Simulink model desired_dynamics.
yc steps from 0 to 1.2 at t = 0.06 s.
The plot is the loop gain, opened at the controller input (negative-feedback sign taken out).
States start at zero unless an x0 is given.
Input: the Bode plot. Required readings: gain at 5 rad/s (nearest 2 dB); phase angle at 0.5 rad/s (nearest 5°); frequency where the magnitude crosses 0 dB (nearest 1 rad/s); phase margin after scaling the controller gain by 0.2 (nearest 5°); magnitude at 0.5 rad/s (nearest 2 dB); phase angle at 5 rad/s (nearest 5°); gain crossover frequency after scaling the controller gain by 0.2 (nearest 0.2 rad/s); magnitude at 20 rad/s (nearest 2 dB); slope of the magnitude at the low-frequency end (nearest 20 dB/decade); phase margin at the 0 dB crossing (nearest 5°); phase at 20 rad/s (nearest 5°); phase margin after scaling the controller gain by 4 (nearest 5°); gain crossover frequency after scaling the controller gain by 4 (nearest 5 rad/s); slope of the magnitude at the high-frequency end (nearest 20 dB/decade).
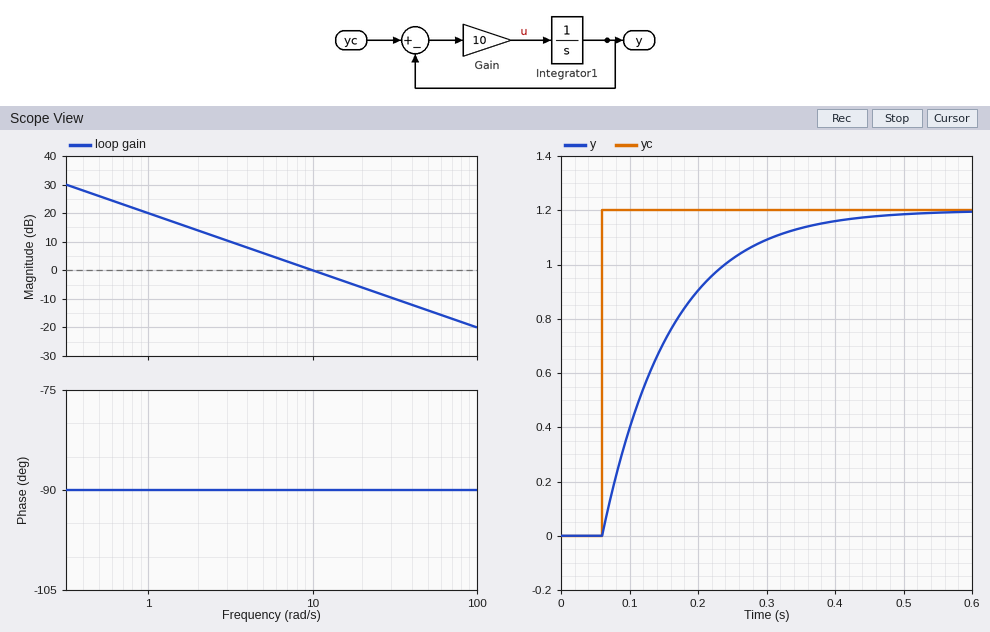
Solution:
6 dB
-90°
10 rad/s
90°
26 dB
-90°
2.0 rad/s
-6 dB
-20 dB/decade
90°
-90°
90°
40 rad/s
-20 dB/decade
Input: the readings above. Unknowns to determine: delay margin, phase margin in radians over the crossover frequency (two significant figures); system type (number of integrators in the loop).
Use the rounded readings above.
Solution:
0.16 s
1
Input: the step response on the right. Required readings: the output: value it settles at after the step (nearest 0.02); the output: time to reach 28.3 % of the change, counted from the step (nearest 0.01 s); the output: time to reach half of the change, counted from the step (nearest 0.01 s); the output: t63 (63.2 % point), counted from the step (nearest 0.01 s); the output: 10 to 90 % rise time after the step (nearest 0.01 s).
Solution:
1.20
0.03 s
0.07 s
0.10 s
0.22 s
